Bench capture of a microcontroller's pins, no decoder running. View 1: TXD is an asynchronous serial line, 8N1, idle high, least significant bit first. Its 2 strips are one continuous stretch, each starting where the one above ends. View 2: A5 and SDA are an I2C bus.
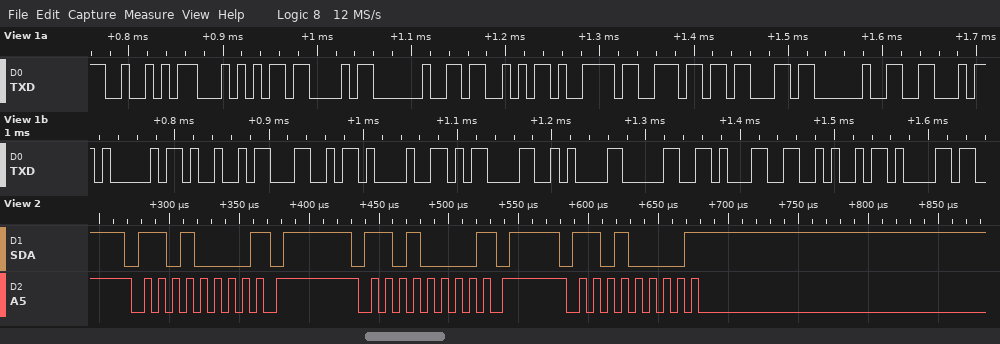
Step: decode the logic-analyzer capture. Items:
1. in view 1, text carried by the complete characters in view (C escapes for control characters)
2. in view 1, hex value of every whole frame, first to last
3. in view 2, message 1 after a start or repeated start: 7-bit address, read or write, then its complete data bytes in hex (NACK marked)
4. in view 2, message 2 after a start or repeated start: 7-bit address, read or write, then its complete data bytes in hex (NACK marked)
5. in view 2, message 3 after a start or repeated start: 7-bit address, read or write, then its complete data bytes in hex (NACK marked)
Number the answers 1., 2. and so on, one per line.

1. "RTC Sync FAIL!\r\n01Ja"
2. 52 54 43 20 53 79 6E 63 20 46 41 49 4C 21 0D 0A 30 31 4A 61
3. 0x68 write NACK
4. 0x68 write NACK
5. 0x68 write NACK
